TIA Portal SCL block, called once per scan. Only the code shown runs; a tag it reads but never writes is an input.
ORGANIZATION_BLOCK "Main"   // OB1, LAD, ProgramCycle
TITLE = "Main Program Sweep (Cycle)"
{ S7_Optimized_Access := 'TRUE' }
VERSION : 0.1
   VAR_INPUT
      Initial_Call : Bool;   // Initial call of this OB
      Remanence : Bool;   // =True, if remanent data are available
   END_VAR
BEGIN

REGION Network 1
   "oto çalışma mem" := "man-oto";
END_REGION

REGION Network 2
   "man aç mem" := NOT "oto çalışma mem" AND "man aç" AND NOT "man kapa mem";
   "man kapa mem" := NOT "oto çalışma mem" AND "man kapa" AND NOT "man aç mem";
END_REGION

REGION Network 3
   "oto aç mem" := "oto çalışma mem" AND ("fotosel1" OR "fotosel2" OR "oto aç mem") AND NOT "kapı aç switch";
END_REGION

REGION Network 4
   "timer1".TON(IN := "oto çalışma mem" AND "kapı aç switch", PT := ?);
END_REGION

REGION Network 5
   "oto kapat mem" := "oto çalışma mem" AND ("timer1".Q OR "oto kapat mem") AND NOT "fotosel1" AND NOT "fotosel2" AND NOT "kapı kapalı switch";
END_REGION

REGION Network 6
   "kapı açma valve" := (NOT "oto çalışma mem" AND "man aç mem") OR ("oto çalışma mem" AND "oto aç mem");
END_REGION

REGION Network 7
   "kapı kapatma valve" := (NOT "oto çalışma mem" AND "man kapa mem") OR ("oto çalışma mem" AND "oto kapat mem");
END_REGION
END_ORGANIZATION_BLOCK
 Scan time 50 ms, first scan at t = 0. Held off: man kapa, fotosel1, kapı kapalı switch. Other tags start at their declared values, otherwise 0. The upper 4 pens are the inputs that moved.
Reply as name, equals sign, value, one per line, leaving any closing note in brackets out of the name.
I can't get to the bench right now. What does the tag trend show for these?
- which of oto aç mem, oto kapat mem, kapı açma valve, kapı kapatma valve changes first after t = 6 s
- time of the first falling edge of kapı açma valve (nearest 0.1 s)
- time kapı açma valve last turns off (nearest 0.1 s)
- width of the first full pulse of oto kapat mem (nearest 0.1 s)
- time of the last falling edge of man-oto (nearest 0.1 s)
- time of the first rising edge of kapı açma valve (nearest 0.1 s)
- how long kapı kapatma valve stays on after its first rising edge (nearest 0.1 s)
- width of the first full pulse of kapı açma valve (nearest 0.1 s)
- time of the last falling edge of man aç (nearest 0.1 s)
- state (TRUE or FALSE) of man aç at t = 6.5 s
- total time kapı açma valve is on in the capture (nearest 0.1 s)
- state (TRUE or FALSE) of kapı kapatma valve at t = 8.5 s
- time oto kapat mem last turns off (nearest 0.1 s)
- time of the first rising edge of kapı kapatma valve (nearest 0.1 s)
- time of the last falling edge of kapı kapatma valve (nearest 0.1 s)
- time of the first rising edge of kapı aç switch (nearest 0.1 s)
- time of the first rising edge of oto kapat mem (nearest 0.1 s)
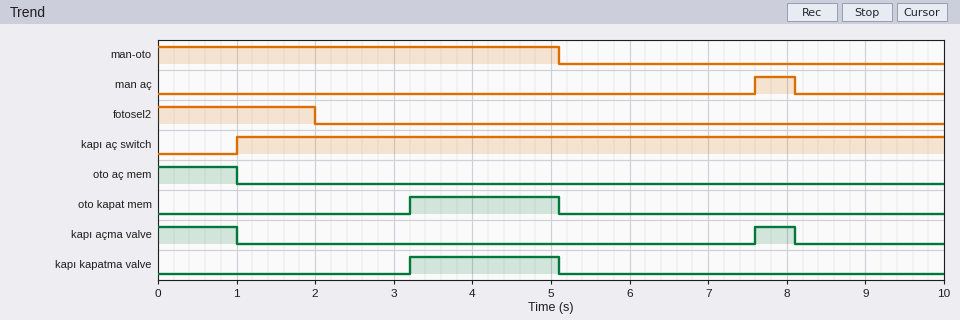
which of oto aç mem, oto kapat mem, kapı açma valve, kapı kapatma valve changes first after t = 6 s = kapı açma valve
time of the first falling edge of kapı açma valve = 1.0 s
time kapı açma valve last turns off = 8.1 s
width of the first full pulse of oto kapat mem = 1.9 s
time of the last falling edge of man-oto = 5.1 s
time of the first rising edge of kapı açma valve = 7.6 s
how long kapı kapatma valve stays on after its first rising edge = 1.9 s
width of the first full pulse of kapı açma valve = 0.5 s
time of the last falling edge of man aç = 8.1 s
state (TRUE or FALSE) of man aç at t = 6.5 s = FALSE
total time kapı açma valve is on in the capture = 1.5 s
state (TRUE or FALSE) of kapı kapatma valve at t = 8.5 s = FALSE
time oto kapat mem last turns off = 5.1 s
time of the first rising edge of kapı kapatma valve = 3.2 s
time of the last falling edge of kapı kapatma valve = 5.1 s
time of the first rising edge of kapı aç switch = 1.0 s
time of the first rising edge of oto kapat mem = 3.2 s
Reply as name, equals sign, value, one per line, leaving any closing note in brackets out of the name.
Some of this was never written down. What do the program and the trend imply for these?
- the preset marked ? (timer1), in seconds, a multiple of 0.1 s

the preset marked ? (timer1), in seconds, a multiple of 0.1 s = 2.2 s
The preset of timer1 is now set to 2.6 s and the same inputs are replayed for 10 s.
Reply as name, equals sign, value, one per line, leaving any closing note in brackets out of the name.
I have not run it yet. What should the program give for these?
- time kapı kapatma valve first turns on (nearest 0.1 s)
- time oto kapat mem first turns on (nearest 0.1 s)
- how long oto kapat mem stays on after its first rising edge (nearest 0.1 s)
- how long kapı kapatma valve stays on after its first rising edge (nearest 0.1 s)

time kapı kapatma valve first turns on = 3.6 s
time oto kapat mem first turns on = 3.6 s
how long oto kapat mem stays on after its first rising edge = 1.5 s
how long kapı kapatma valve stays on after its first rising edge = 1.5 s
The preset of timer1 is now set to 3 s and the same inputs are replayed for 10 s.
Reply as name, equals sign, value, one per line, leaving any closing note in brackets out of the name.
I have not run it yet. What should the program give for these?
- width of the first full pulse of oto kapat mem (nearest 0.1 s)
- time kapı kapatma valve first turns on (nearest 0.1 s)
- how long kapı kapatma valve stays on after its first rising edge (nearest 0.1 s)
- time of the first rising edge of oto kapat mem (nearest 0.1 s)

width of the first full pulse of oto kapat mem = 1.1 s
time kapı kapatma valve first turns on = 4.0 s
how long kapı kapatma valve stays on after its first rising edge = 1.1 s
time of the first rising edge of oto kapat mem = 4.0 s
